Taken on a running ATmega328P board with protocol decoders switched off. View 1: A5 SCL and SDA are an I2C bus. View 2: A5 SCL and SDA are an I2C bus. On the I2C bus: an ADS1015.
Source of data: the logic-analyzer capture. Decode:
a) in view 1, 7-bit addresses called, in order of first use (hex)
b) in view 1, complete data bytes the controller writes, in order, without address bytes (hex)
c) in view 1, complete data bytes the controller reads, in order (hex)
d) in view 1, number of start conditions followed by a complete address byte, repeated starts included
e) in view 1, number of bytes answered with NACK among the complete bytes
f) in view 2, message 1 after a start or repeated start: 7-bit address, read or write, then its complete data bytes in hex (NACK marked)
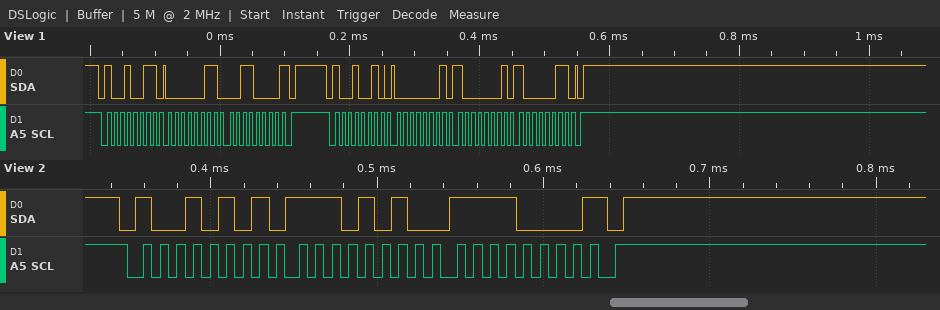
0x49
01 81 83
03 30
2
1
0x4A read: EA F0 NACK
